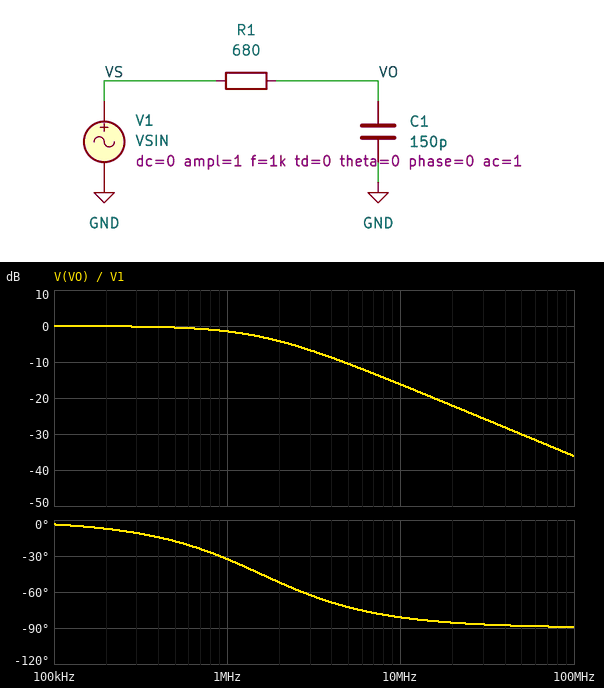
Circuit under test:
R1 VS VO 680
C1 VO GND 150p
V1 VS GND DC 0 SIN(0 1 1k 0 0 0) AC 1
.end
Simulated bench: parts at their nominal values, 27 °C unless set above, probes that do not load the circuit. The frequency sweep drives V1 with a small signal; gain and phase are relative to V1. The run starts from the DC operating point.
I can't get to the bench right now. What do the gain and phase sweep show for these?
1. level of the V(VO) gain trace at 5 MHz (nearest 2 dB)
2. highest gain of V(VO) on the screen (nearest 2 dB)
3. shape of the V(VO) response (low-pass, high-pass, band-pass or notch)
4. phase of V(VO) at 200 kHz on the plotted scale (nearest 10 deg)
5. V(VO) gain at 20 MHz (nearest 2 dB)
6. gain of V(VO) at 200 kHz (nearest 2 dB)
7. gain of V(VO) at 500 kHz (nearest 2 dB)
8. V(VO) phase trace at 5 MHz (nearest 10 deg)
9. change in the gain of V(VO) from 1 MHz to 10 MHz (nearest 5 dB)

-10 dB
0 dB
low-pass
-10 deg
-22 dB
0 dB
0 dB
-70 deg
-15 dB
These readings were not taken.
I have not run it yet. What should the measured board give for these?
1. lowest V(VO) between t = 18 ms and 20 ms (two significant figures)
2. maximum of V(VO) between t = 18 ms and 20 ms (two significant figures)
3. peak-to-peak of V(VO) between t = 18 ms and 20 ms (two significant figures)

-1.0 V
1.0 V
2.0 V
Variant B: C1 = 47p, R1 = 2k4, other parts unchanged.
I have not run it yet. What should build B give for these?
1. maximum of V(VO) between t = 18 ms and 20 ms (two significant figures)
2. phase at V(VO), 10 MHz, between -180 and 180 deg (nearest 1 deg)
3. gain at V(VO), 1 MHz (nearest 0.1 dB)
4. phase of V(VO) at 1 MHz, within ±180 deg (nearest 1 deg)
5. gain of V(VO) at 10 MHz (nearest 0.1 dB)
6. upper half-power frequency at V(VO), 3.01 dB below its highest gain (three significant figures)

1.0 V
-82 deg
-1.8 dB
-35 deg
-17.1 dB
1.41 MHz
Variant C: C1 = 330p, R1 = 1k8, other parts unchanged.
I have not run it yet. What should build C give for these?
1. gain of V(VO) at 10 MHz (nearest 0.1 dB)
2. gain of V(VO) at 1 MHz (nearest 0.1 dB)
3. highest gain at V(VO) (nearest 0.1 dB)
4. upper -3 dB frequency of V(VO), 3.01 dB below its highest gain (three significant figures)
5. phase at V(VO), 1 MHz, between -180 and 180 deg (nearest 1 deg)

-31.4 dB
-11.7 dB
0 dB
268 kHz
-75 deg
